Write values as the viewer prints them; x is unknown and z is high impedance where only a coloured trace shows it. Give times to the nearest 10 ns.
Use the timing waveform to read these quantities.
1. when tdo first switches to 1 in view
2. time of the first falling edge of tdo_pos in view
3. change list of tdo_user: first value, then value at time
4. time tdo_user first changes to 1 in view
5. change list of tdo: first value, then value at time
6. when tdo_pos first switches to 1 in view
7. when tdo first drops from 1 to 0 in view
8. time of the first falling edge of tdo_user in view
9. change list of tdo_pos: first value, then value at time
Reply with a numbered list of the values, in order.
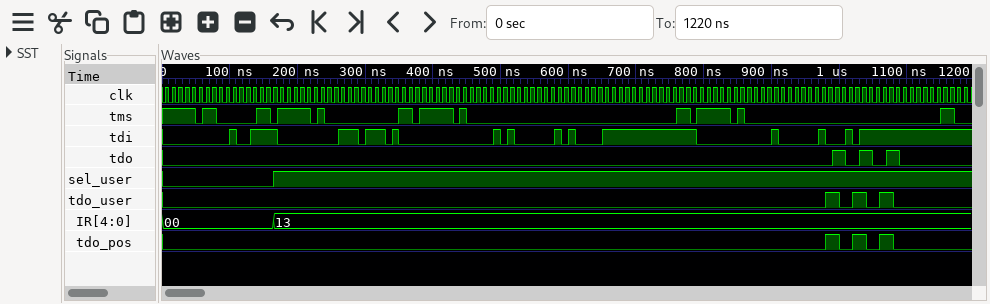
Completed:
1. 990 ns
2. 1000 ns
3. 0, 1 at 980 ns, 0 at 1000 ns, 1 at 1020 ns, 0 at 1040 ns, 1 at 1060 ns, 0 at 1080 ns
4. 980 ns
5. 0, 1 at 990 ns, 0 at 1010 ns, 1 at 1030 ns, 0 at 1050 ns, 1 at 1070 ns, 0 at 1090 ns
6. 980 ns
7. 1010 ns
8. 1000 ns
9. 0, 1 at 980 ns, 0 at 1000 ns, 1 at 1020 ns, 0 at 1040 ns, 1 at 1060 ns, 0 at 1080 ns
